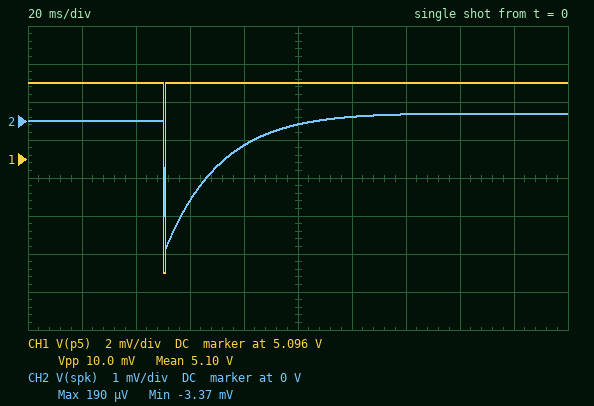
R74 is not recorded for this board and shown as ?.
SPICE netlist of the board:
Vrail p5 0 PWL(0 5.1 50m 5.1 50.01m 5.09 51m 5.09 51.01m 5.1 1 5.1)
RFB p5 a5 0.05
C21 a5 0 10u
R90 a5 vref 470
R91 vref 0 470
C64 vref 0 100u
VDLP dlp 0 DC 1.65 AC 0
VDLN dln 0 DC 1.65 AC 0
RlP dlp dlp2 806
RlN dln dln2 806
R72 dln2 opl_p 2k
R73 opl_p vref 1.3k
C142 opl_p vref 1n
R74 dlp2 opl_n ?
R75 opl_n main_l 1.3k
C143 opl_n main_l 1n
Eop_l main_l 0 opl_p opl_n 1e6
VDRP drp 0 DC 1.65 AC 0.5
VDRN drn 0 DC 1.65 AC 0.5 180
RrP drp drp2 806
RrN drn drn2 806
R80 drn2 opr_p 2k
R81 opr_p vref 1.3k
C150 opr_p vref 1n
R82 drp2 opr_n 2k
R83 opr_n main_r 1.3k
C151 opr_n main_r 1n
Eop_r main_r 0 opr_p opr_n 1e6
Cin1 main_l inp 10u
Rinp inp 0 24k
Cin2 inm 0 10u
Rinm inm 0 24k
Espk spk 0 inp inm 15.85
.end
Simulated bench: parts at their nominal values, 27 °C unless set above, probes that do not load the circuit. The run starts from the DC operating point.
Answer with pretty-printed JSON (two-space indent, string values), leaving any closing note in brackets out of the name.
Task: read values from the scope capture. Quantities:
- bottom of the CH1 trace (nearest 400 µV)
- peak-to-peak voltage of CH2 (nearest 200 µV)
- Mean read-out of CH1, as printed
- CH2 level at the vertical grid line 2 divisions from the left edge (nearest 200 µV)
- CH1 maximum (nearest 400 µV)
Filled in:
{
  "bottom of the CH1 trace": "5.0900 V",
  "peak-to-peak voltage of CH2": "3.6 mV",
  "Mean read-out of CH1, as printed": "5.10 V",
  "CH2 level at the vertical grid line 2 divisions from the left edge": "0 V",
  "CH1 maximum": "5.1000 V"
}
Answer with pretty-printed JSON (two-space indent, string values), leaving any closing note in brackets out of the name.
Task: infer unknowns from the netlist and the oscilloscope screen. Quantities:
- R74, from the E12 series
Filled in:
{
  "R74, from the E12 series": "1.8 kΩ"
}
